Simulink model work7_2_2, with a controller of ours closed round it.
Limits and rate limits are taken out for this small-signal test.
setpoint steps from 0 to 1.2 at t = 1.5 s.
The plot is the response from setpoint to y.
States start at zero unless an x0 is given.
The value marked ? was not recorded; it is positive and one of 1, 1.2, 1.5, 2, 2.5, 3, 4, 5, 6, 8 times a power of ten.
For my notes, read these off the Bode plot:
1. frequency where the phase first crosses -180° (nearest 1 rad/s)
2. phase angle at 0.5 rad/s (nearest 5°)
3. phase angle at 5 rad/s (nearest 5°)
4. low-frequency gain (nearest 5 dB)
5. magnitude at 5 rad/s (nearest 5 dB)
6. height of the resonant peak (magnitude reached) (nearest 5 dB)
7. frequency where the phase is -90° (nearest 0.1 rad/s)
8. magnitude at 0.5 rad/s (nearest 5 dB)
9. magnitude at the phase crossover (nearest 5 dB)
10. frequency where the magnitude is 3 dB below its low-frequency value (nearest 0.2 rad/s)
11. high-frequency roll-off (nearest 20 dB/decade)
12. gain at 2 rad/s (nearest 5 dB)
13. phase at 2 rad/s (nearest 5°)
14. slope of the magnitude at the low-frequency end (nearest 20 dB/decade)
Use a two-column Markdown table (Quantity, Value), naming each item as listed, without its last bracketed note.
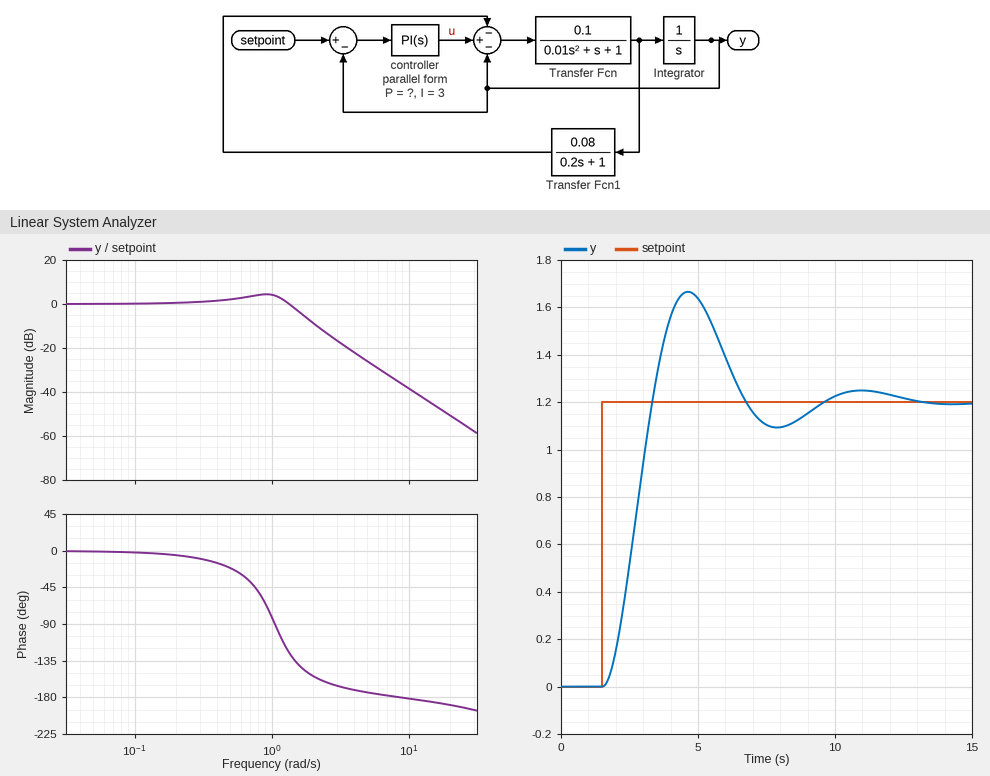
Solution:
| Quantity | Value |
|---|---|
| frequency where the phase first crosses -180° | 9 rad/s |
| phase angle at 0.5 rad/s | -20° |
| phase angle at 5 rad/s | -175° |
| low-frequency gain | 0 dB |
| magnitude at 5 rad/s | -25 dB |
| height of the resonant peak (magnitude reached) | 5 dB |
| frequency where the phase is -90° | 1.1 rad/s |
| magnitude at 0.5 rad/s | 0 dB |
| magnitude at the phase crossover | -35 dB |
| frequency where the magnitude is 3 dB below its low-frequency value | 1.6 rad/s |
| high-frequency roll-off | -40 dB/decade |
| gain at 2 rad/s | -10 dB |
| phase at 2 rad/s | -155° |
| slope of the magnitude at the low-frequency end | 0 dB/decade |
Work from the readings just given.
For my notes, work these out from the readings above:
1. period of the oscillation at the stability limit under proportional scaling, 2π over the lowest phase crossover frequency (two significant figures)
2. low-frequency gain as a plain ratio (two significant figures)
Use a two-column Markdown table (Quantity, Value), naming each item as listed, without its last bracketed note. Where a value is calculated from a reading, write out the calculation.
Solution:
| Quantity | Value |
|---|---|
| period of the oscillation at the stability limit under proportional scaling, 2π over the lowest phase crossover frequency | 2π / 9 = 0.70 s |
| low-frequency gain as a plain ratio | 10^(0 / 20) = 1.0 |
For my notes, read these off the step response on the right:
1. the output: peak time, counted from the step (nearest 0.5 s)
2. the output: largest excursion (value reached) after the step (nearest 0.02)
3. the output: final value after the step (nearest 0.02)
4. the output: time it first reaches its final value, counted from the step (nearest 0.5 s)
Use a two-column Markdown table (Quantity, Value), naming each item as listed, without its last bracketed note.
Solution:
| Quantity | Value |
|---|---|
| the output: peak time, counted from the step | 3.0 s |
| the output: largest excursion (value reached) after the step | 1.66 |
| the output: final value after the step | 1.20 |
| the output: time it first reaches its final value, counted from the step | 2.0 s |
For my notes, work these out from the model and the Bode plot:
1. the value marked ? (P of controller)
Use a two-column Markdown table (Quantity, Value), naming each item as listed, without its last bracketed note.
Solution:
| Quantity | Value |
|---|---|
| the value marked ? | 12 |
